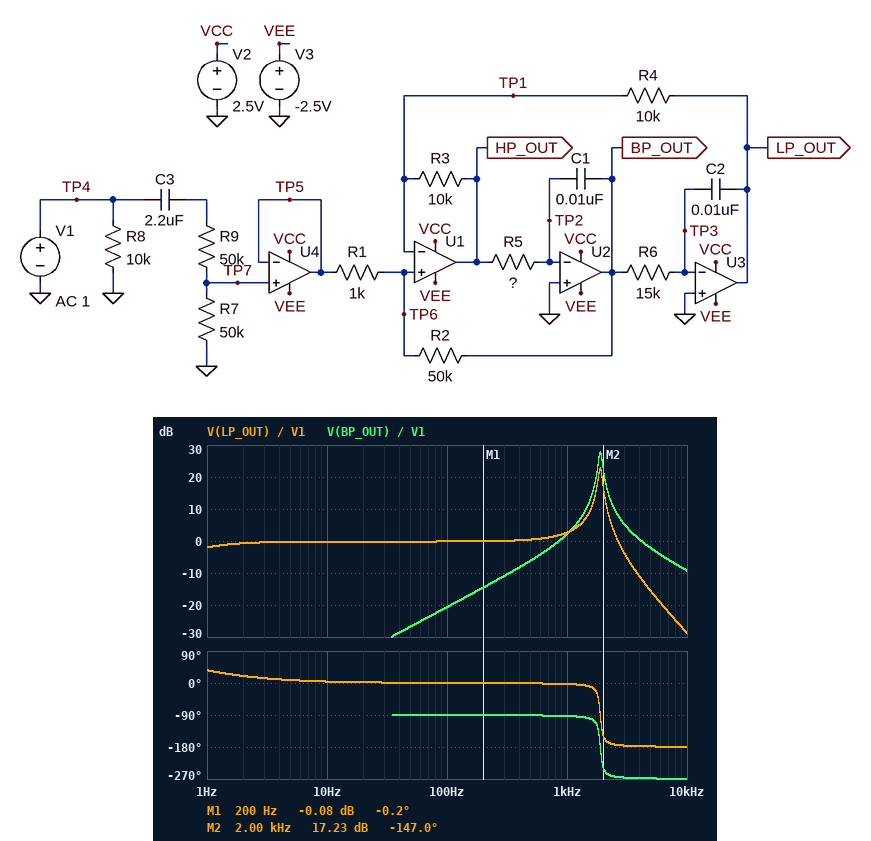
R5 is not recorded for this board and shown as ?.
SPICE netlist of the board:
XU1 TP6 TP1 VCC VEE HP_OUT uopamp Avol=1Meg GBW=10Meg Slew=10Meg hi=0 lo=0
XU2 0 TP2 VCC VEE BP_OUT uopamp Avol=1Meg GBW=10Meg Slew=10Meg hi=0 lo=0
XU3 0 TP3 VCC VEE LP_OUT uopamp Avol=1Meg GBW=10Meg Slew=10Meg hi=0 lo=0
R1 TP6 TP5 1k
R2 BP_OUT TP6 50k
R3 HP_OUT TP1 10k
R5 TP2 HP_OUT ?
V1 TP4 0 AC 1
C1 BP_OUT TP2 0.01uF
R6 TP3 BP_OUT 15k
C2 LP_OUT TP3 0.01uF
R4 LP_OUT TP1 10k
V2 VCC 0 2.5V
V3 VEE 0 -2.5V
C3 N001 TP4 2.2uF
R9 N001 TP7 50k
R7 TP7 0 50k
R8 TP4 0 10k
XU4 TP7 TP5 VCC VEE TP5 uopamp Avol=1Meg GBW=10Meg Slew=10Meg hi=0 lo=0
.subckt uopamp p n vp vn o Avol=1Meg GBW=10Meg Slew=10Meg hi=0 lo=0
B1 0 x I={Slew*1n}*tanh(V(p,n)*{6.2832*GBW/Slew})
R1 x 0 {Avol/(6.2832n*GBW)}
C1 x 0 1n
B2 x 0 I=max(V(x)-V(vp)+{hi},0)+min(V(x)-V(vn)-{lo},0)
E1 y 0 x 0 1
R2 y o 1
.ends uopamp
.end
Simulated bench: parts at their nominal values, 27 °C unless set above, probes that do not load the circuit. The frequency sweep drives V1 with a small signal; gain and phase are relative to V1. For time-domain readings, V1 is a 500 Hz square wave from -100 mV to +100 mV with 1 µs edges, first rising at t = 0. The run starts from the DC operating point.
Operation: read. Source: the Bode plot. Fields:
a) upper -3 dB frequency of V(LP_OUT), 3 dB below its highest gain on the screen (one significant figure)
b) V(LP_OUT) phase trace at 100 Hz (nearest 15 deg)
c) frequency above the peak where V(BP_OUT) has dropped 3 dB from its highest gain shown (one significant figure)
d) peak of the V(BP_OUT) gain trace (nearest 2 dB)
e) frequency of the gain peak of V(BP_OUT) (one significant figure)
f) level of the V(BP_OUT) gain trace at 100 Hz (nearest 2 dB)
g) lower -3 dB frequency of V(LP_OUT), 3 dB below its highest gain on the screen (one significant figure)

2 kHz
0 deg
2 kHz
28 dB
2 kHz
-20 dB
2 kHz
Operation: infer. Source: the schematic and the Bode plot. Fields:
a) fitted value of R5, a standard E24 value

4.7 kΩ
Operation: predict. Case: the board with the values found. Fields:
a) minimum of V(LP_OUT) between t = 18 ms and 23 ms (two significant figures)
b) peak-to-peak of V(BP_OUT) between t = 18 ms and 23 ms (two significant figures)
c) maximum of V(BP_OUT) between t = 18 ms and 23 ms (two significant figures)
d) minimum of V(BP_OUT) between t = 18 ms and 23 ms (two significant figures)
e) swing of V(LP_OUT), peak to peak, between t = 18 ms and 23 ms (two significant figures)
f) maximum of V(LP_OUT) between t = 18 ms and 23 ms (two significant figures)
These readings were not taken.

-120 mV
430 mV
210 mV
-210 mV
420 mV
300 mV
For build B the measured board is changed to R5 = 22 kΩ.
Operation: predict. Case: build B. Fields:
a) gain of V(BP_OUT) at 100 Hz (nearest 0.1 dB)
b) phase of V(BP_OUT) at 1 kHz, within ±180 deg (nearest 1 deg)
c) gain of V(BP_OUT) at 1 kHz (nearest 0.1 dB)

-20.6 dB
97 deg
9.6 dB
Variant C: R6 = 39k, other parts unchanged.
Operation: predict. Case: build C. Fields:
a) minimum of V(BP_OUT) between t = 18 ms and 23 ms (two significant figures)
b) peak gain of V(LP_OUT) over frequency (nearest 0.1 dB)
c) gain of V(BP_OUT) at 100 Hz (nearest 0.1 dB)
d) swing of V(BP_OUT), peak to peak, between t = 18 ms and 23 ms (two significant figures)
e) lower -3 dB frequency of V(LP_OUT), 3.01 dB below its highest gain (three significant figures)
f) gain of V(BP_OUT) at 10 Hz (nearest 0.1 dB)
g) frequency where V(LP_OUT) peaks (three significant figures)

-350 mV
18.8 dB
-12.3 dB
710 mV
1.10 kHz
-32.4 dB
1.17 kHz
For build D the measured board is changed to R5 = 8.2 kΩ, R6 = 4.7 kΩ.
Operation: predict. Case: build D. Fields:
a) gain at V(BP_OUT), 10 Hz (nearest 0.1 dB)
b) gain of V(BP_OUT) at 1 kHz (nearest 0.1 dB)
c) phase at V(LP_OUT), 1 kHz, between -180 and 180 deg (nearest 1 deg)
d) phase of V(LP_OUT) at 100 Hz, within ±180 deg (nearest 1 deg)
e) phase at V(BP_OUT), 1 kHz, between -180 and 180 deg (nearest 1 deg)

-50.8 dB
-9.3 dB
-1 deg
0 deg
-91 deg
